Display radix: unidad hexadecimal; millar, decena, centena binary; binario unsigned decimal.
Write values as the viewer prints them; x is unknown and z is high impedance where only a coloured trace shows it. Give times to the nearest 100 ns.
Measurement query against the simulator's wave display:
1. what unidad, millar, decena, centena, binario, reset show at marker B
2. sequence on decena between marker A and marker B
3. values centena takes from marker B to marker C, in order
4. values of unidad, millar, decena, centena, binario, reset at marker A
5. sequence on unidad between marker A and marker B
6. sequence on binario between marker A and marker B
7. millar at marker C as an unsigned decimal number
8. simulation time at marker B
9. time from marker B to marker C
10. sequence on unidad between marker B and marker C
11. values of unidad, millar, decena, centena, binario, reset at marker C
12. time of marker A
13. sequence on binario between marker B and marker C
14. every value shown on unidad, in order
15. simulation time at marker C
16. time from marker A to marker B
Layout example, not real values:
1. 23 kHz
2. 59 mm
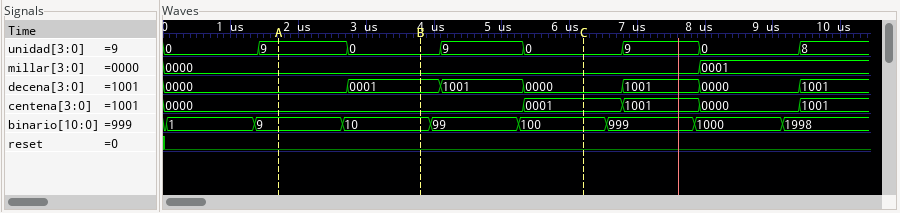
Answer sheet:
1. unidad=0, millar=0000, decena=0001, centena=0000, binario=10, reset=0
2. 0000, 0001
3. 0000, 0001
4. unidad=9, millar=0000, decena=0000, centena=0000, binario=9, reset=0
5. 9, 0
6. 9, 10
7. 0
8. 3800 ns
9. 2400 ns
10. 0, 9, 0
11. unidad=0, millar=0000, decena=0000, centena=0001, binario=100, reset=0
12. 1700 ns
13. 10, 99, 100
14. 0, 9, 0, 9, 0, 9, 0, 8
15. 6200 ns
16. 2100 ns
